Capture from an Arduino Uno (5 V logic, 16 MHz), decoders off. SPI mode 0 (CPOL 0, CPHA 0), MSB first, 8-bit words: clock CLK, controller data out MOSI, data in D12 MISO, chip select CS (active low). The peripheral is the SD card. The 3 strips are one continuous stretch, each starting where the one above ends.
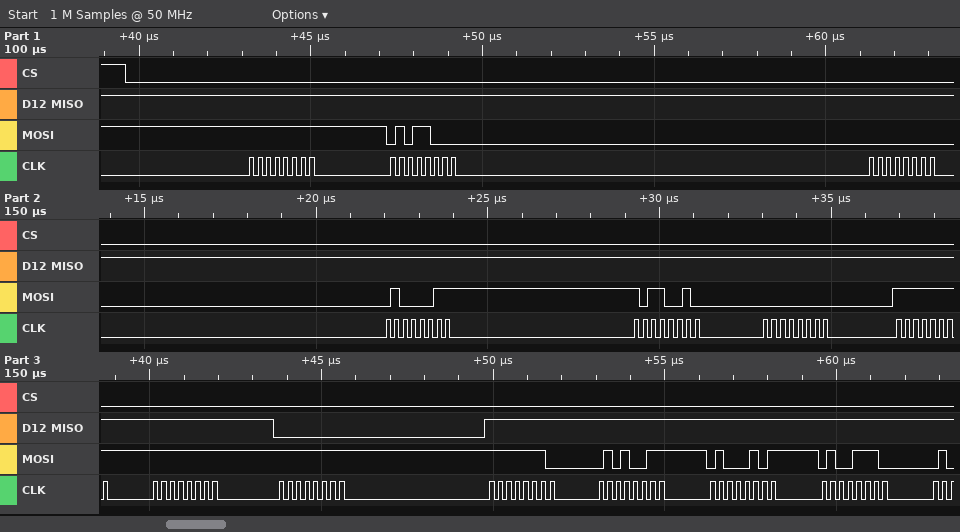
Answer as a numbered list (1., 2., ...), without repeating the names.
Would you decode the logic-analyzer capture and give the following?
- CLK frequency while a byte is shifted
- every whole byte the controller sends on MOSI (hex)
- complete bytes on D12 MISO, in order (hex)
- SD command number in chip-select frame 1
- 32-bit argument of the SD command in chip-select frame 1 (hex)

1. 4 MHz
2. 0xFF 0x58 0x00 0x43 0xB2 0x00 0xFF 0xFF 0xFF 0xFE 0x53 0x45 0x4E
3. 0xFF 0xFF 0xFF 0xFF 0xFF 0xFF 0xFF 0xFF 0x00 0xFF 0xFF 0xFF 0xFF
4. CMD24
5. 0x0043B200
